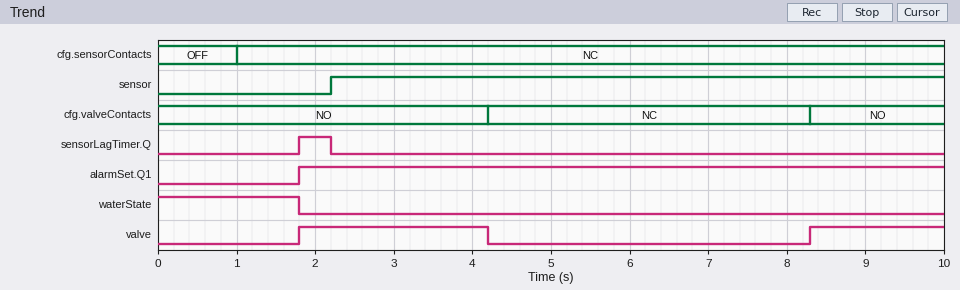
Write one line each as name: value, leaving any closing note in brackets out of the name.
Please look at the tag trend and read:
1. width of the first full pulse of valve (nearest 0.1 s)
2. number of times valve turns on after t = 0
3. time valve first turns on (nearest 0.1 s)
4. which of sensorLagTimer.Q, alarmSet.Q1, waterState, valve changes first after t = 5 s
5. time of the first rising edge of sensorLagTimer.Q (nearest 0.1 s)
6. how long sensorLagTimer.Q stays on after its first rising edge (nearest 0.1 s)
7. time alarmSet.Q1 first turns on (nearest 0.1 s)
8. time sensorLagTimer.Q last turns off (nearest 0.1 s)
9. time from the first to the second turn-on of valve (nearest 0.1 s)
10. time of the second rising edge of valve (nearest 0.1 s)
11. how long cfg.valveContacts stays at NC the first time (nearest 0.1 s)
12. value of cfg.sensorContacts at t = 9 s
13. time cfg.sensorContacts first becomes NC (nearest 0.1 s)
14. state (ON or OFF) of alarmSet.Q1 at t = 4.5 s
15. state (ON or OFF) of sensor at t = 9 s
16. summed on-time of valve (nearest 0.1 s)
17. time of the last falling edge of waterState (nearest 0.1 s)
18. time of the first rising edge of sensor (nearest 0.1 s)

width of the first full pulse of valve: 2.4 s
number of times valve turns on after t = 0: 2
time valve first turns on: 1.8 s
which of sensorLagTimer.Q, alarmSet.Q1, waterState, valve changes first after t = 5 s: valve
time of the first rising edge of sensorLagTimer.Q: 1.8 s
how long sensorLagTimer.Q stays on after its first rising edge: 0.4 s
time alarmSet.Q1 first turns on: 1.8 s
time sensorLagTimer.Q last turns off: 2.2 s
time from the first to the second turn-on of valve: 6.5 s
time of the second rising edge of valve: 8.3 s
how long cfg.valveContacts stays at NC the first time: 4.1 s
value of cfg.sensorContacts at t = 9 s: NC
time cfg.sensorContacts first becomes NC: 1.0 s
state (ON or OFF) of alarmSet.Q1 at t = 4.5 s: ON
state (ON or OFF) of sensor at t = 9 s: ON
summed on-time of valve: 4.1 s
time of the last falling edge of waterState: 1.8 s
time of the first rising edge of sensor: 2.2 s
